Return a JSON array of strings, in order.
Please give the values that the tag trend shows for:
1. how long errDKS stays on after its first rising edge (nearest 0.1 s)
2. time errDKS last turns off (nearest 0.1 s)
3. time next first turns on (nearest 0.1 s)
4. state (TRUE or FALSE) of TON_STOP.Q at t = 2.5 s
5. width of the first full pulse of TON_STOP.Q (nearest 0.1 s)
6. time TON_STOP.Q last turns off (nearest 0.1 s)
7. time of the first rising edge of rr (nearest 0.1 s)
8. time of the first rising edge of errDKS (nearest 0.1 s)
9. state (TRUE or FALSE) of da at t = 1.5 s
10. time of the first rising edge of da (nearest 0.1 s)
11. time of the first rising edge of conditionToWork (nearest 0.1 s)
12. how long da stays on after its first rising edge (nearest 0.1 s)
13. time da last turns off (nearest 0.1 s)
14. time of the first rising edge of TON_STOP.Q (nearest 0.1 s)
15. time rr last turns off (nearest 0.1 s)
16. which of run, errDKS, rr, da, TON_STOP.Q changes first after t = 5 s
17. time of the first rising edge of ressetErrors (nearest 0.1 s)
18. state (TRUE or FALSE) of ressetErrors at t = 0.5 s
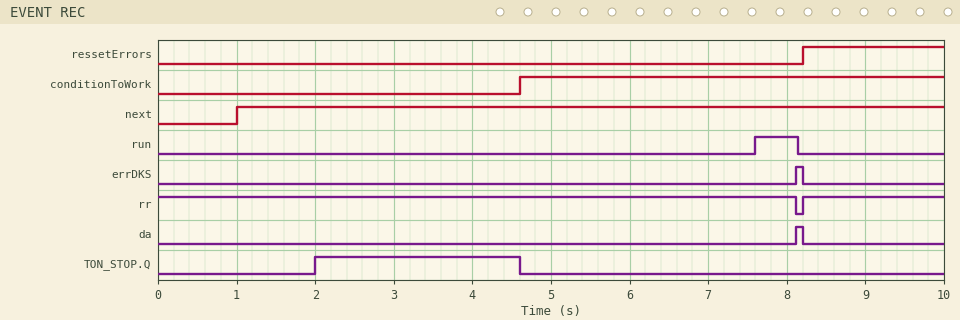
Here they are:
["0.1 s", "8.2 s", "1.0 s", "TRUE", "2.6 s", "4.6 s", "8.2 s", "8.1 s", "FALSE", "8.1 s", "4.6 s", "0.1 s", "8.2 s", "2.0 s", "8.1 s", "run", "8.2 s", "FALSE"]
